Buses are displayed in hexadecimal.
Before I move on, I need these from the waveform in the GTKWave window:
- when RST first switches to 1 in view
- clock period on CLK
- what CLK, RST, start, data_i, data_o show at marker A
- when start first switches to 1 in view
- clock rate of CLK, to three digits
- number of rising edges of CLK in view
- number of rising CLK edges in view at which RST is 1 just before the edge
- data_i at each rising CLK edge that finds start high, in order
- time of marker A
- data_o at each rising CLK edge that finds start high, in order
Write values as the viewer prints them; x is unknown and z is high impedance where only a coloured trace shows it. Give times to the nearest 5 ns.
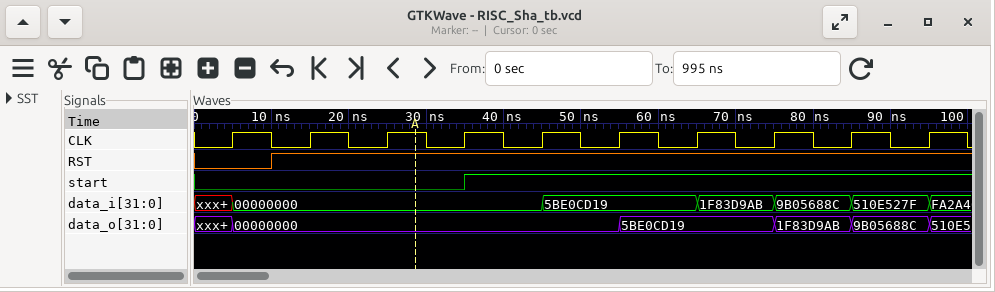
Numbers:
10 ns
10 ns
CLK=1, RST=1, start=0, data_i=00000000, data_o=00000000
35 ns
100 MHz
10
9
00000000, 5BE0CD19, 5BE0CD19, 1F83D9AB, 9B05688C, 510E527F
30 ns
00000000, 00000000, 5BE0CD19, 5BE0CD19, 1F83D9AB, 9B05688C
